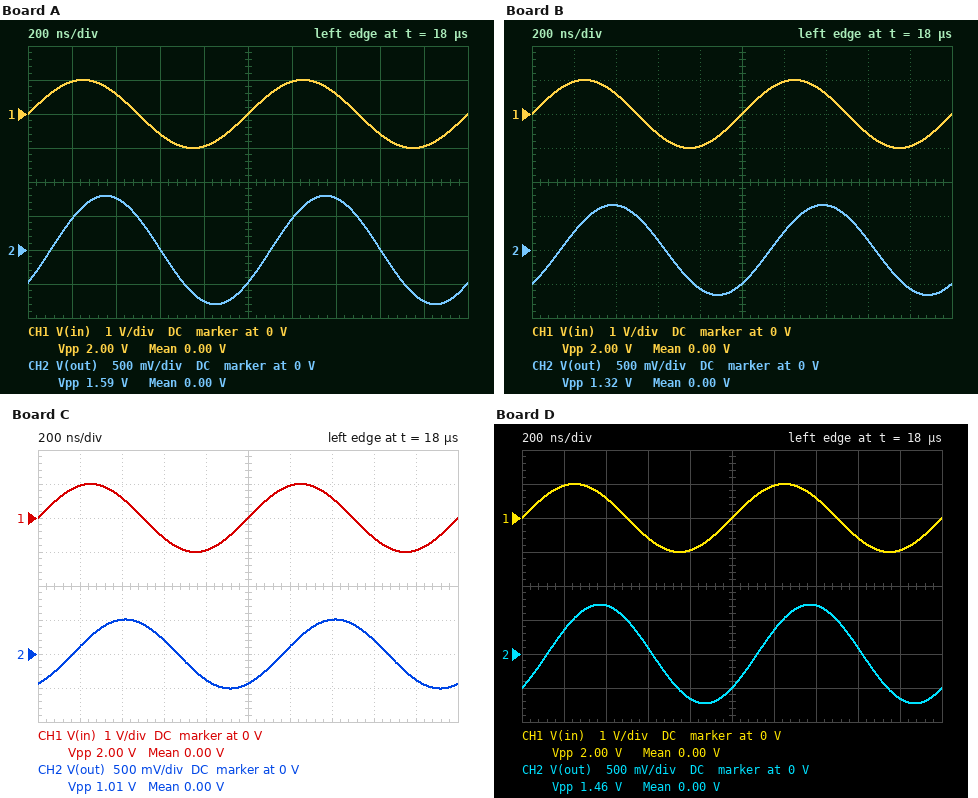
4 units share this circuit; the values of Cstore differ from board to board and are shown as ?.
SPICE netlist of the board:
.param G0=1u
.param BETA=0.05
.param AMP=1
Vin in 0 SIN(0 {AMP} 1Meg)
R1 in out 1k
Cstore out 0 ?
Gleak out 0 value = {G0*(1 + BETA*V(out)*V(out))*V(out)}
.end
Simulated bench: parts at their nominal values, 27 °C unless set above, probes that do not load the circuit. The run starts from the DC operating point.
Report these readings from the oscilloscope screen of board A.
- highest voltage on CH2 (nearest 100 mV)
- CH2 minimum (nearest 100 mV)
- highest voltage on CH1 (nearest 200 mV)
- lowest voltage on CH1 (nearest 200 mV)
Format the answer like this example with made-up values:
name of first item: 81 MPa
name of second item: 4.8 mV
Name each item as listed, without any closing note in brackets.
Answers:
highest voltage on CH2: 800 mV
CH2 minimum: -800 mV
highest voltage on CH1: 1.0 V
lowest voltage on CH1: -1.0 V
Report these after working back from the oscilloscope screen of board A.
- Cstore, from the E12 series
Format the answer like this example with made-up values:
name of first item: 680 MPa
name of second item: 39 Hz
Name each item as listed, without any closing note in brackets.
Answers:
Cstore, from the E12 series: 120 pF
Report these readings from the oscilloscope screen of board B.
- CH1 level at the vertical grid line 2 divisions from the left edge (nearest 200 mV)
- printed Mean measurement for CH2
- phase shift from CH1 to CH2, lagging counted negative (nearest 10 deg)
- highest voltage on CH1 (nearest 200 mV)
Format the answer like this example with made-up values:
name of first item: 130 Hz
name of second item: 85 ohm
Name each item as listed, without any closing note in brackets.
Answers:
CH1 level at the vertical grid line 2 divisions from the left edge: 600 mV
printed Mean measurement for CH2: 0.00 V
phase shift from CH1 to CH2, lagging counted negative: -50 deg
highest voltage on CH1: 1.0 V
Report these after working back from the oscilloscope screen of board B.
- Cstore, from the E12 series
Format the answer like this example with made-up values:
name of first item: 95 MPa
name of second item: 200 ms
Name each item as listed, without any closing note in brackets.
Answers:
Cstore, from the E12 series: 180 pF
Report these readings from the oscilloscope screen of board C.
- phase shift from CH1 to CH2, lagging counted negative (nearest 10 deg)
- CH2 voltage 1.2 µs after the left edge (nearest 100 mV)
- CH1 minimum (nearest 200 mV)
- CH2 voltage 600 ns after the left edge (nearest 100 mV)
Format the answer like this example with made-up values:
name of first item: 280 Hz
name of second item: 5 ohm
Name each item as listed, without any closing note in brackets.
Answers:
phase shift from CH1 to CH2, lagging counted negative: -60 deg
CH2 voltage 1.2 µs after the left edge: 100 mV
CH1 minimum: -1.0 V
CH2 voltage 600 ns after the left edge: 200 mV
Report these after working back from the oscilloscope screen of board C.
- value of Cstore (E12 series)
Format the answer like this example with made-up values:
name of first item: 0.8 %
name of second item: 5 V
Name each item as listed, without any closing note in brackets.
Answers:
value of Cstore: 270 pF
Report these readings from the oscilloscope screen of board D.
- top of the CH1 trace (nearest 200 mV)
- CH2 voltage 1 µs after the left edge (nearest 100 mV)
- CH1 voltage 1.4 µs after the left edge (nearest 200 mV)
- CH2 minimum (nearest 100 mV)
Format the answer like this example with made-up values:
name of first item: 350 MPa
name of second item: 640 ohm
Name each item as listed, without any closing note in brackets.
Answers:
top of the CH1 trace: 1.0 V
CH2 voltage 1 µs after the left edge: -500 mV
CH1 voltage 1.4 µs after the left edge: 600 mV
CH2 minimum: -700 mV
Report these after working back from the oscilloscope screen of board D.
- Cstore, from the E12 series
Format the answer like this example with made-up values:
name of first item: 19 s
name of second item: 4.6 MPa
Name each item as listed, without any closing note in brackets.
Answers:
Cstore, from the E12 series: 150 pF
